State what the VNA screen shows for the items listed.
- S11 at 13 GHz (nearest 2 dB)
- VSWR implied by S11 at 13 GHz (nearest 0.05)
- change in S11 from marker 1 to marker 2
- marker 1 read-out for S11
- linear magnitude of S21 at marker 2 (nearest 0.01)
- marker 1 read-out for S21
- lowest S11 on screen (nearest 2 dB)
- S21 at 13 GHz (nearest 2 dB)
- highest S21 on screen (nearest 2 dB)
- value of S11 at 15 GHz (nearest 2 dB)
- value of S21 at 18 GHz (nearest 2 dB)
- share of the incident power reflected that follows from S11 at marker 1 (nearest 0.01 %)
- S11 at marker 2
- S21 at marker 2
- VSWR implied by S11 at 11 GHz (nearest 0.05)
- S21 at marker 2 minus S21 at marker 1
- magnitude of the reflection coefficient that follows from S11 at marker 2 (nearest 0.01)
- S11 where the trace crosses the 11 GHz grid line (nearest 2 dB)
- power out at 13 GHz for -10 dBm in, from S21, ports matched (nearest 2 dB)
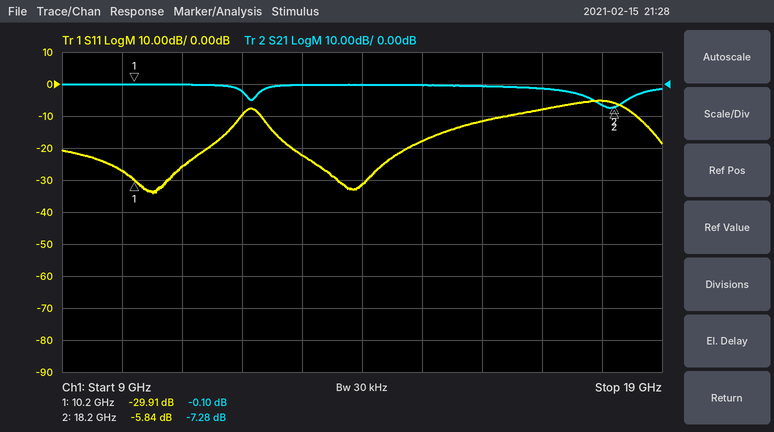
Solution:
-22 dB
1.15
24.07 dB
-29.91 dB
0.43
-0.10 dB
-34 dB
0 dB
0 dB
-18 dB
-6 dB
0.10 %
-5.84 dB
-7.28 dB
1.10
-7.18 dB
0.51
-26 dB
-10 dBm
